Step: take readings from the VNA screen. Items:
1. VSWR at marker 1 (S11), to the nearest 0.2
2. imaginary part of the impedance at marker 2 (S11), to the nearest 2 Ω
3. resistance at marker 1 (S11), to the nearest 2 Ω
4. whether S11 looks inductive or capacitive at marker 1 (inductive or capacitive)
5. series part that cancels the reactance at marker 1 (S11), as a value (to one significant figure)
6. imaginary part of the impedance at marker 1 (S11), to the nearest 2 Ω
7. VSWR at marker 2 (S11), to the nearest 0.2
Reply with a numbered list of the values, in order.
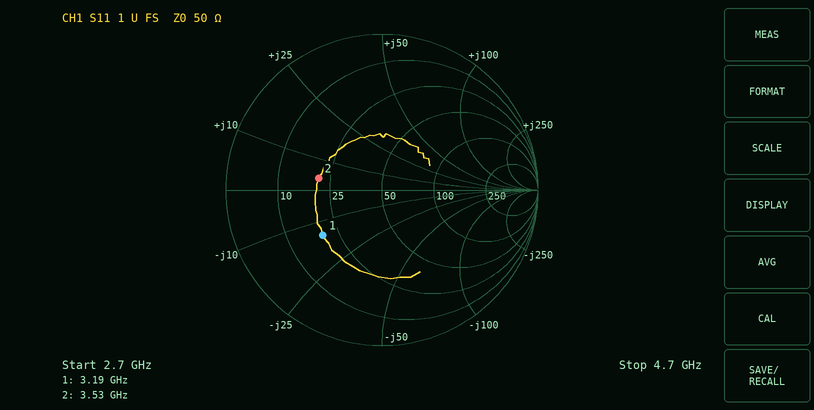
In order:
1. 2.8
2. +4 Ω
3. 20 Ω
4. capacitive
5. 700 pH
6. -14 Ω
7. 2.4
